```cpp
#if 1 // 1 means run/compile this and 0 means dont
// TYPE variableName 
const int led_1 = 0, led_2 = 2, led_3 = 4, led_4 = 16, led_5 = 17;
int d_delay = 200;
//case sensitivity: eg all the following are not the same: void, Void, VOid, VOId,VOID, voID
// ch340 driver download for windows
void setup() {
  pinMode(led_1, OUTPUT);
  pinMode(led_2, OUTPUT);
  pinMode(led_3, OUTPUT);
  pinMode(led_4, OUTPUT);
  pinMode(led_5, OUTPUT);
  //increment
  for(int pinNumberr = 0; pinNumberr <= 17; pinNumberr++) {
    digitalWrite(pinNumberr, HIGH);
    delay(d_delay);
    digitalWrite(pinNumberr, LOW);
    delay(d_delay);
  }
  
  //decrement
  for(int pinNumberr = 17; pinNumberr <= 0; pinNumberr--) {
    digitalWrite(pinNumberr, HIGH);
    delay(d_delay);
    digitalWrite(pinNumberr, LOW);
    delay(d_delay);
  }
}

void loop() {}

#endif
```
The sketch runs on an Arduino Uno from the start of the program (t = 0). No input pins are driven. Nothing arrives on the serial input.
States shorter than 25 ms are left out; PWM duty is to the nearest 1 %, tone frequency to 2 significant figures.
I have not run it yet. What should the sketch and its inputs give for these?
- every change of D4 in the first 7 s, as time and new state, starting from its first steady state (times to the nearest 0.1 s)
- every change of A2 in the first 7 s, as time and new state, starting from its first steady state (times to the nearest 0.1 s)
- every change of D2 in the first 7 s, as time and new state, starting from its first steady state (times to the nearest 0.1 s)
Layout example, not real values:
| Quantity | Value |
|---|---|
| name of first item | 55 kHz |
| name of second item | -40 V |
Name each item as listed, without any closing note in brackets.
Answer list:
| Quantity | Value |
|---|---|
| every change of D4 in the first 7 s, as time and new state, starting from its first steady state | 0 s low; 1.6 s high; 1.8 s low |
| every change of A2 in the first 7 s, as time and new state, starting from its first steady state | 0 s low; 6.4 s high; 6.6 s low |
| every change of D2 in the first 7 s, as time and new state, starting from its first steady state | 0 s low; 0.8 s high; 1 s low |
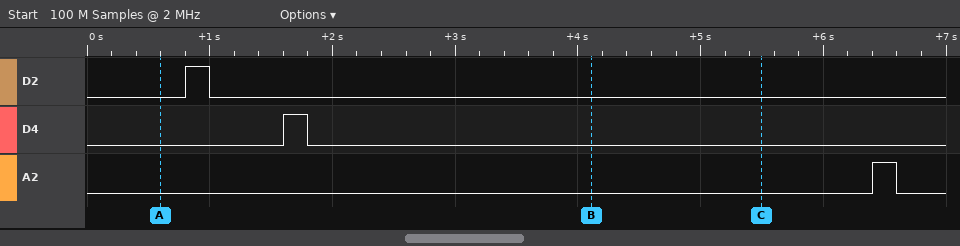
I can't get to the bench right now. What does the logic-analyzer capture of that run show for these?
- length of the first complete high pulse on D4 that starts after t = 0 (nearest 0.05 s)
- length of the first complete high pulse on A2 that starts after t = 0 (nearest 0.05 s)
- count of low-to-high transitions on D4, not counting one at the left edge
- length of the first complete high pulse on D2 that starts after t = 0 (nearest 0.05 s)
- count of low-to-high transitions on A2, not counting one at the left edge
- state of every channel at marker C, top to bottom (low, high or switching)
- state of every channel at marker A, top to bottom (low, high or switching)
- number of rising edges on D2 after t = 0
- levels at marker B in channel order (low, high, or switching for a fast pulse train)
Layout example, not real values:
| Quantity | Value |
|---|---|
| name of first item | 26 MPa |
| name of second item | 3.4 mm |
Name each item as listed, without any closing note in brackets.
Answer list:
| Quantity | Value |
|---|---|
| length of the first complete high pulse on D4 that starts after t = 0 | 0.20 s |
| length of the first complete high pulse on A2 that starts after t = 0 | 0.20 s |
| count of low-to-high transitions on D4, not counting one at the left edge | 1 |
| length of the first complete high pulse on D2 that starts after t = 0 | 0.20 s |
| count of low-to-high transitions on A2, not counting one at the left edge | 1 |
| state of every channel at marker C, top to bottom | D2 low, D4 low, A2 low |
| state of every channel at marker A, top to bottom | D2 low, D4 low, A2 low |
| number of rising edges on D2 after t = 0 | 1 |
| levels at marker B in channel order | D2 low, D4 low, A2 low |
